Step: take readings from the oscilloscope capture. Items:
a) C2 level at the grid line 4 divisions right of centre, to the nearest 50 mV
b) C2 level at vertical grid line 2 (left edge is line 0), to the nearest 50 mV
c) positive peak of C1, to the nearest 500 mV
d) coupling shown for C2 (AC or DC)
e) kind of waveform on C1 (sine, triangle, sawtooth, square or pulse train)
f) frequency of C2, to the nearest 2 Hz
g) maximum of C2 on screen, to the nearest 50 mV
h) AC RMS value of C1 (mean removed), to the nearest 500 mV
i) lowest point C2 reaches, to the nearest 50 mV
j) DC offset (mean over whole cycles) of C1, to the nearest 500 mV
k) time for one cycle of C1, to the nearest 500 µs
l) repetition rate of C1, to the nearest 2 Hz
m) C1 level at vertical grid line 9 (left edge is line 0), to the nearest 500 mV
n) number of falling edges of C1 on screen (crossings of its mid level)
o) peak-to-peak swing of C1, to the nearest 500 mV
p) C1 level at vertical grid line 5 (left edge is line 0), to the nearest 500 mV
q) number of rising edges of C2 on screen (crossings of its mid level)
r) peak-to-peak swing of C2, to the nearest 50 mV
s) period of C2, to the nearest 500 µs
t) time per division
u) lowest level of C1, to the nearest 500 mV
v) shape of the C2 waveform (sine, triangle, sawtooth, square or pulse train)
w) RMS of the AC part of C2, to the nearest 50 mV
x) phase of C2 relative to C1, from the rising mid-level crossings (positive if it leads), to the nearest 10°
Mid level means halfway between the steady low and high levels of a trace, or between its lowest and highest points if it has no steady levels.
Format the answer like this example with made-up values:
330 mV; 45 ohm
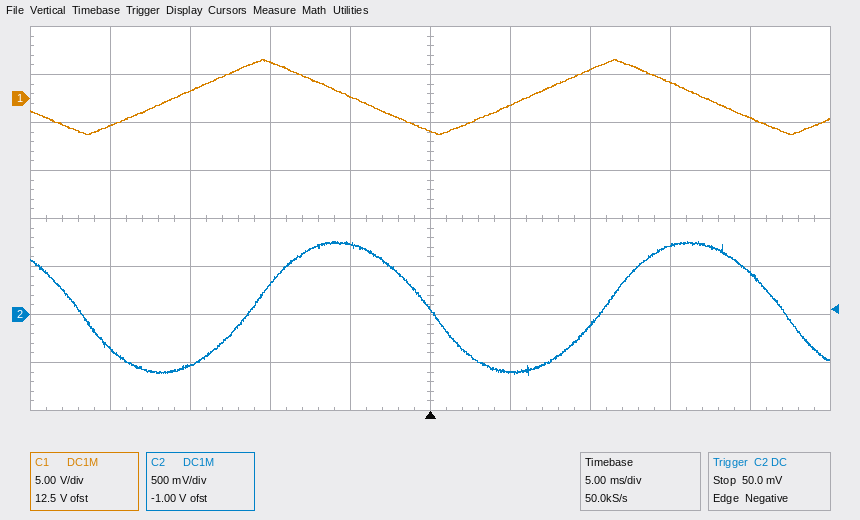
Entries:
450 mV; -550 mV; 4.0 V; DC; triangle; 46 Hz; 750 mV; 2.5 V; -650 mV; 0.0 V; 22.0 ms; 46 Hz; -2.0 V; 2; 8.0 V; -3.5 V; 2; 1.40 V; 22.0 ms; 5 ms; -4.0 V; sine; 500 mV; -80°
